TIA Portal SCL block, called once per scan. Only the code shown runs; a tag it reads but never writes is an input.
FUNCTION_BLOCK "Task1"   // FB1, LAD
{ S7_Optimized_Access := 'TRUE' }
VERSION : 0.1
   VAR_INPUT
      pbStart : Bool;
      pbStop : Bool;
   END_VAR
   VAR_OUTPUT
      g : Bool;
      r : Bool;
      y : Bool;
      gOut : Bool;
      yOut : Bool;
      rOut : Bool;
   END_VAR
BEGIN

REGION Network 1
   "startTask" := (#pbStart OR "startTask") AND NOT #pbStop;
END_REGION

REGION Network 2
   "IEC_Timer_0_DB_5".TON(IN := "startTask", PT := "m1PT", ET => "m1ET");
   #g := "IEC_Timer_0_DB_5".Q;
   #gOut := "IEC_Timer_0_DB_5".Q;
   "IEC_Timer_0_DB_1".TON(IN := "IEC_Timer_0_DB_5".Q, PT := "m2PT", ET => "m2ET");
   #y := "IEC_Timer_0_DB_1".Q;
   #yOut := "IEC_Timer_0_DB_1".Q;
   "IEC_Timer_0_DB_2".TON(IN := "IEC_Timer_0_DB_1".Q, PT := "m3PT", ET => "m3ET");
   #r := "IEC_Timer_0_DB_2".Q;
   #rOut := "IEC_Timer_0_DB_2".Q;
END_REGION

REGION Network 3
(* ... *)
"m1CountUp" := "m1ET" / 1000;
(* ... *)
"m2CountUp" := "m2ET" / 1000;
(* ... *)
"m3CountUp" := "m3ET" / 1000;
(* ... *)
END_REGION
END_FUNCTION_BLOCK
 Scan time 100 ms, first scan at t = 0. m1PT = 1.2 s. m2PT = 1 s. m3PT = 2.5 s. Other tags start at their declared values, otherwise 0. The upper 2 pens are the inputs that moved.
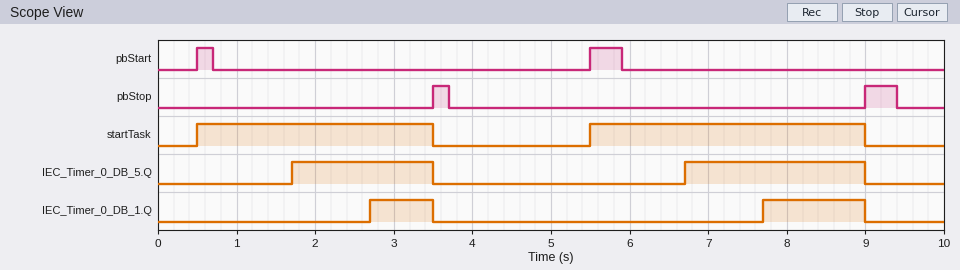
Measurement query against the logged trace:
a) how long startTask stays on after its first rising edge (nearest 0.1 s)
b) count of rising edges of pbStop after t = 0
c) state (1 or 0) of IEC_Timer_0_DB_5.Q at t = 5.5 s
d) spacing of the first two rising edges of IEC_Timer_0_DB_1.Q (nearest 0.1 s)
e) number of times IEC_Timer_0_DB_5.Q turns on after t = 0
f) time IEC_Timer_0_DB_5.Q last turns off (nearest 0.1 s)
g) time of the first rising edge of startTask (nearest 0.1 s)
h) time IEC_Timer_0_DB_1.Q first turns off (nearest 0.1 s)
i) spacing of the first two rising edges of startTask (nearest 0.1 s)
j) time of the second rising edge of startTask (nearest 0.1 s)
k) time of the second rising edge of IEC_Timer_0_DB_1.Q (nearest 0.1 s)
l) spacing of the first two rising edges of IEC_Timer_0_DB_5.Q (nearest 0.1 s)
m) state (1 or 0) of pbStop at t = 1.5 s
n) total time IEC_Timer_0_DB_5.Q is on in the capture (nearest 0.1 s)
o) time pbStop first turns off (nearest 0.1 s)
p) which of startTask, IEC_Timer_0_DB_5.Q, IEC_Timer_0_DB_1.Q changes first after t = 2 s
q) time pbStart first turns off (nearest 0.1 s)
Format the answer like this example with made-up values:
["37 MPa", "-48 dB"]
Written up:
["3.0 s", "2", "0", "5.0 s", "2", "9.0 s", "0.5 s", "3.5 s", "5.0 s", "5.5 s", "7.7 s", "5.0 s", "0", "4.1 s", "3.7 s", "IEC_Timer_0_DB_1.Q", "0.7 s"]
